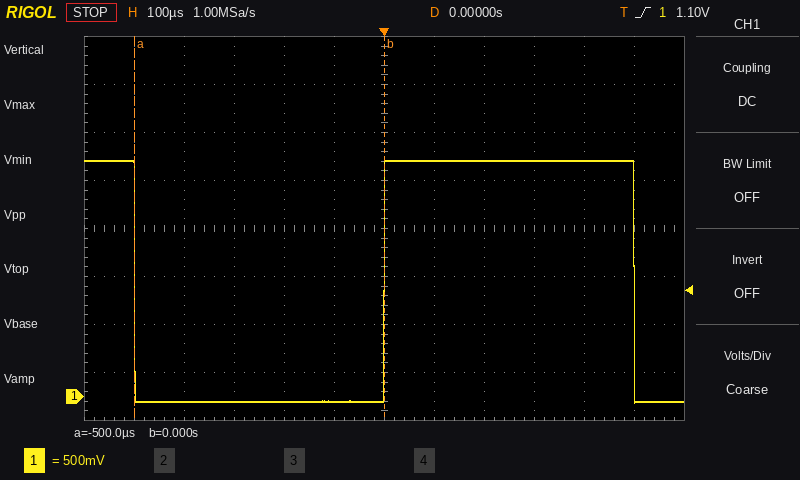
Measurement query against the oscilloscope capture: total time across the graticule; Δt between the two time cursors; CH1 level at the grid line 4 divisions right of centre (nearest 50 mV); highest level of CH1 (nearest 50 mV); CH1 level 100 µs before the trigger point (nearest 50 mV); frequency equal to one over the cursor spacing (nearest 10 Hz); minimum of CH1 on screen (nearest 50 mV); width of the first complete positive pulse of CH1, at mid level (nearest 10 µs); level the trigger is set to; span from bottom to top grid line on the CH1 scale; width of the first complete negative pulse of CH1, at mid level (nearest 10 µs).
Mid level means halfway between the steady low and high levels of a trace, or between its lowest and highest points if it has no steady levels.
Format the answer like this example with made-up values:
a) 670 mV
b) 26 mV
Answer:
a) 1.2 ms
b) 500 µs
c) 2.45 V
d) 2.45 V
e) -50 mV
f) 2.00 kHz
g) -50 mV
h) 500 µs
i) 1.10 V
j) 4 V
k) 500 µs
